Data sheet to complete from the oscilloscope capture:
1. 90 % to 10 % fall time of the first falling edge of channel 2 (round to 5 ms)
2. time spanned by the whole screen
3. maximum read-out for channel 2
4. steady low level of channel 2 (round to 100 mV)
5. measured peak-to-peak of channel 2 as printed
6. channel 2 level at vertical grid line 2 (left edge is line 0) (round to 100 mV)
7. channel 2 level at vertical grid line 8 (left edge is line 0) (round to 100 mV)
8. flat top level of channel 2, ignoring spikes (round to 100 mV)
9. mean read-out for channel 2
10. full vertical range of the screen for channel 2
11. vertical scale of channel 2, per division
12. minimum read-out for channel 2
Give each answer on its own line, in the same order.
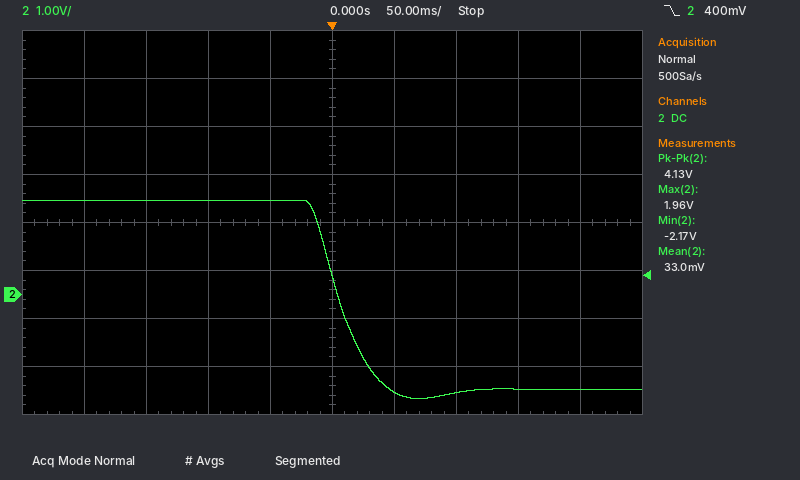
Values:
45 ms
500 ms
1.96 V
-2.0 V
4.13 V
2.0 V
-2.0 V
2.0 V
33.0 mV
8 V
1 V
-2.17 V
